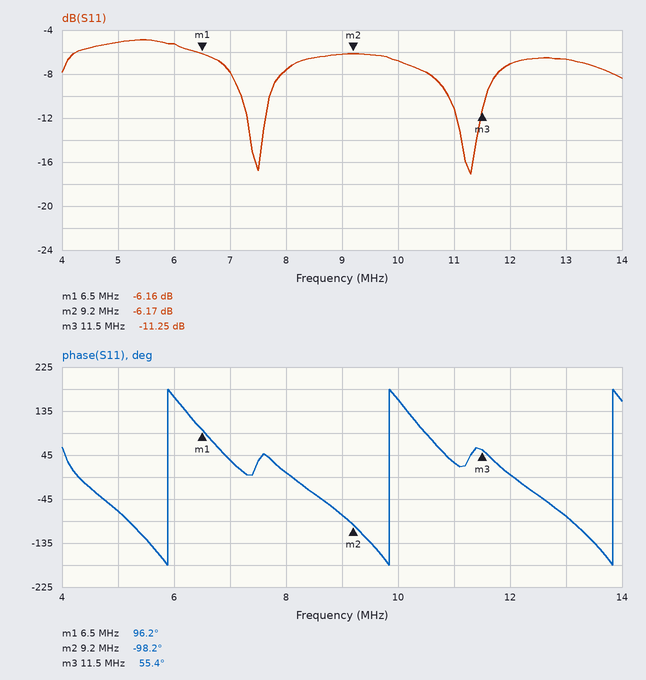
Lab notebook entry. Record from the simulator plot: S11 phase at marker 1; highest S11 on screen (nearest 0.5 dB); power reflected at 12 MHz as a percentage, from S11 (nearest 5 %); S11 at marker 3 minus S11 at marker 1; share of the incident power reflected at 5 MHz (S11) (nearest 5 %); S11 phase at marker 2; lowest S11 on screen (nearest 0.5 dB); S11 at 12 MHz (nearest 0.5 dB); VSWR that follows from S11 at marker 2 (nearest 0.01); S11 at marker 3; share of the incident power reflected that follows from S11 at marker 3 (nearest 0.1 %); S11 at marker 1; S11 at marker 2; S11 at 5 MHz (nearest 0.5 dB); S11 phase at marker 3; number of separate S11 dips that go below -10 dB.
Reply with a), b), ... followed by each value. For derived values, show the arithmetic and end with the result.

a) 96.2°
b) -5.0 dB
c) 10^(-7/10) ≈ 20 %
d) -11.25 − (-6.16) = -5.09 dB
e) 10^(-5/10) ≈ 31.6 %, so 30 % to the nearest 5 %
f) -98.2°
g) -17.0 dB
h) -7.0 dB
i) (1 + 0.4915)/(1 − 0.4915) ≈ 2.93
j) -11.25 dB
k) 10^(-11.25/10) ≈ 7.5 %
l) -6.16 dB
m) -6.17 dB
n) -5.0 dB
o) 55.4°
p) 2
